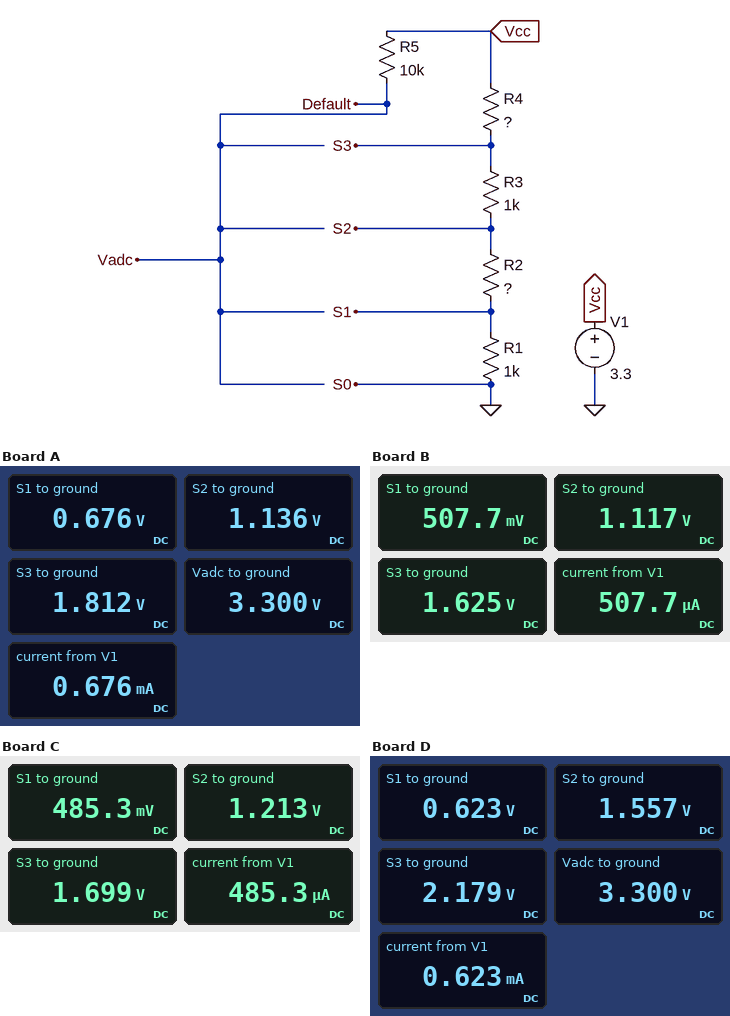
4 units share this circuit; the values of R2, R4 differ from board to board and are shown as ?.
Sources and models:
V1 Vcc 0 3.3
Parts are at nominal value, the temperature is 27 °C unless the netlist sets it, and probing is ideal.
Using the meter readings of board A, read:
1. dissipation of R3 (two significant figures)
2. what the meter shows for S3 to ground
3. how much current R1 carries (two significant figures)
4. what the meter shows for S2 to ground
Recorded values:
460 µW
1.812 V
680 µA
1.136 V
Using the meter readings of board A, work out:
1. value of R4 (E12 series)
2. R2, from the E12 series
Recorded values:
2.2 kΩ
680 Ω
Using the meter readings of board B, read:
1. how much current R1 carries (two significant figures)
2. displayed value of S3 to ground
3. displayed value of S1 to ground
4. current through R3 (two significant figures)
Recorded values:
510 µA
1.625 V
507.7 mV
510 µA
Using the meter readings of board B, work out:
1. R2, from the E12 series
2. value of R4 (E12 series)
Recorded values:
1.2 kΩ
3.3 kΩ
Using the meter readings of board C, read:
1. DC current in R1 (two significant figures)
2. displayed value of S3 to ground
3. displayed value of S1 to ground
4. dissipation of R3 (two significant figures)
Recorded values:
490 µA
1.699 V
485.3 mV
240 µW
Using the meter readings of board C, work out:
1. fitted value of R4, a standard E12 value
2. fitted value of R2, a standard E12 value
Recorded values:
3.3 kΩ
1.5 kΩ
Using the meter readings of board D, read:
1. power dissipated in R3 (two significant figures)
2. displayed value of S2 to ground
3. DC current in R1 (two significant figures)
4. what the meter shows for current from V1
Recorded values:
390 µW
1.557 V
620 µA
0.623 mA
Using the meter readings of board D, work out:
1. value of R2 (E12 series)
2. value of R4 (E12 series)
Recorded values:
1.5 kΩ
1.8 kΩ
